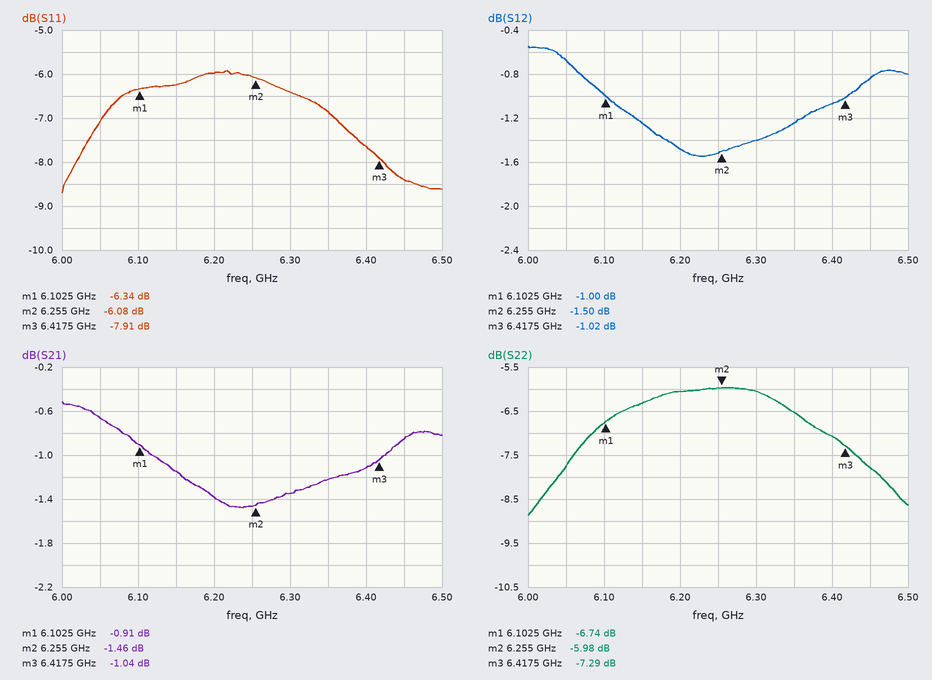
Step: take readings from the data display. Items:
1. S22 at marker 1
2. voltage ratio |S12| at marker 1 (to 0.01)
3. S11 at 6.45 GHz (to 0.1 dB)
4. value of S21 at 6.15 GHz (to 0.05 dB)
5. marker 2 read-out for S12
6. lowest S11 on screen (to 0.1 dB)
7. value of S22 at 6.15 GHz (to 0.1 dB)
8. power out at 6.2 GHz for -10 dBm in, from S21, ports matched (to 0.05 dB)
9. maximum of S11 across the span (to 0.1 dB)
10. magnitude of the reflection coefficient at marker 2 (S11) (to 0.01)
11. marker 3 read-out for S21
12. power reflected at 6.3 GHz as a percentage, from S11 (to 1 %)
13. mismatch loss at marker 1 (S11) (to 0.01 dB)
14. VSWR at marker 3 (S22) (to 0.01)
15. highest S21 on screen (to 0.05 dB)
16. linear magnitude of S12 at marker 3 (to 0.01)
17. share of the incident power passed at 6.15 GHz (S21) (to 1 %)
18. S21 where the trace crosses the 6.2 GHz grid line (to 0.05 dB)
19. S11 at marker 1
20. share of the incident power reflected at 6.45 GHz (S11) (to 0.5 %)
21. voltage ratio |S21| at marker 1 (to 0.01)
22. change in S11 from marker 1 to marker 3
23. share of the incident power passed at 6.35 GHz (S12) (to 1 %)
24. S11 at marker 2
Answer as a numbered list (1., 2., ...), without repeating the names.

1. -6.74 dB
2. 0.89
3. -8.4 dB
4. -1.15 dB
5. -1.50 dB
6. -8.7 dB
7. -6.3 dB
8. -11.40 dBm
9. -5.9 dB
10. 0.50
11. -1.04 dB
12. 23 %
13. 1.15 dB
14. 2.52
15. -0.50 dB
16. 0.89
17. 77 %
18. -1.40 dB
19. -6.34 dB
20. 14.5 %
21. 0.90
22. -1.57 dB
23. 75 %
24. -6.08 dB
